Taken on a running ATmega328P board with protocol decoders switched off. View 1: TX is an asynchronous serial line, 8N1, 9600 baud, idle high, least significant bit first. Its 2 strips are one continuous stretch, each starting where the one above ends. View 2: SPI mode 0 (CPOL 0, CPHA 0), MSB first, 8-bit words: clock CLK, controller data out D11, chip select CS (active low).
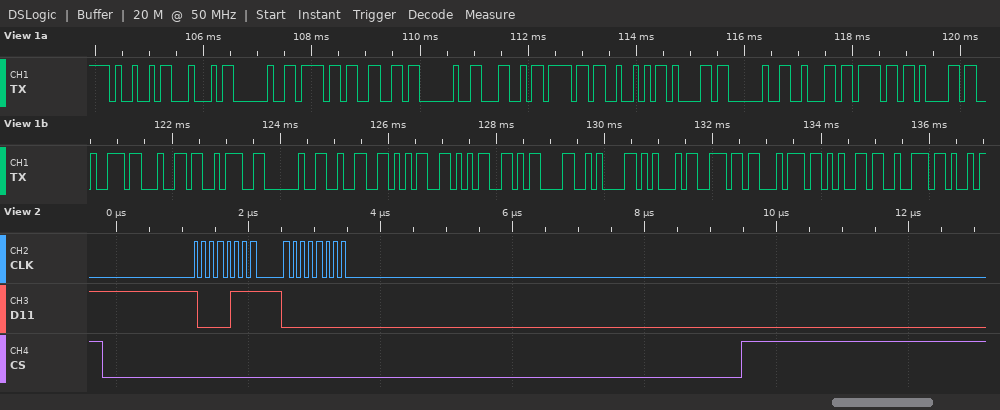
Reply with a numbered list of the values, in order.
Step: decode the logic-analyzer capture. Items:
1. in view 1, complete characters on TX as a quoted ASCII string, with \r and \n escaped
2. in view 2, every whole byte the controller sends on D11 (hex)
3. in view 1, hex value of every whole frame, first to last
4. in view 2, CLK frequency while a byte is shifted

1. "ID of LoRa board: 255\r\nEnter"
2. 87 00
3. 49 44 20 6F 66 20 4C 6F 52 61 20 62 6F 61 72 64 3A 20 32 35 35 0D 0A 45 6E 74 65 72
4. 8 MHz
